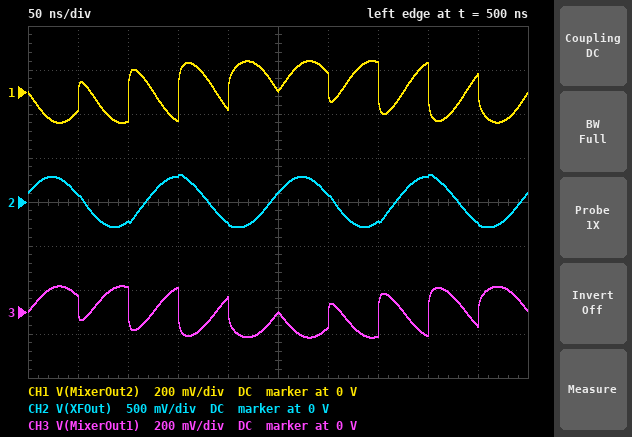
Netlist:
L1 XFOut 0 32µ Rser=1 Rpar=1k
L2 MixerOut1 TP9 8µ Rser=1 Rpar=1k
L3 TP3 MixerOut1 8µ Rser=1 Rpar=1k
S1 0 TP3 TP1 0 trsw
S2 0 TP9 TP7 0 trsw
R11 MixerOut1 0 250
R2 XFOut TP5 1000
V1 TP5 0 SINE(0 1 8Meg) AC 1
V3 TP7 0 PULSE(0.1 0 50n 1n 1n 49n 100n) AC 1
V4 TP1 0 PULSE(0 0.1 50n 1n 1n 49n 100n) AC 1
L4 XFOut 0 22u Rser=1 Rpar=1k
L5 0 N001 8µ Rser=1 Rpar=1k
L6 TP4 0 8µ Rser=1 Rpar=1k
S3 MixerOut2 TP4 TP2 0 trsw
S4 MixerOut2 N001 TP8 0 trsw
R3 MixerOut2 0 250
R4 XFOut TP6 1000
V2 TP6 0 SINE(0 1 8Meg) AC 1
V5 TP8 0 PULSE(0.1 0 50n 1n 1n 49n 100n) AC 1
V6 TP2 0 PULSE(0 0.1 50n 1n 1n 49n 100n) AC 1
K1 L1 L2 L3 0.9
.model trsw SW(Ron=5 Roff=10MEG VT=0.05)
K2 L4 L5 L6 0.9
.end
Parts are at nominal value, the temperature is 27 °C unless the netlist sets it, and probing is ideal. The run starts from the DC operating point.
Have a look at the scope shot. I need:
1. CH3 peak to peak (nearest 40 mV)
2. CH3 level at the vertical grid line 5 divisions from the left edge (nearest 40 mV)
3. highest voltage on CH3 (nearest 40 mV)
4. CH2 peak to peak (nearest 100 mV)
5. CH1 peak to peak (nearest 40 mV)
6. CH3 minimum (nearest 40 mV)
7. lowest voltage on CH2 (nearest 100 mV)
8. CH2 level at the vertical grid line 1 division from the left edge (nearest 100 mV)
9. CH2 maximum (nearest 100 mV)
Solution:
240 mV
0 V
120 mV
600 mV
280 mV
-120 mV
-300 mV
100 mV
300 mV
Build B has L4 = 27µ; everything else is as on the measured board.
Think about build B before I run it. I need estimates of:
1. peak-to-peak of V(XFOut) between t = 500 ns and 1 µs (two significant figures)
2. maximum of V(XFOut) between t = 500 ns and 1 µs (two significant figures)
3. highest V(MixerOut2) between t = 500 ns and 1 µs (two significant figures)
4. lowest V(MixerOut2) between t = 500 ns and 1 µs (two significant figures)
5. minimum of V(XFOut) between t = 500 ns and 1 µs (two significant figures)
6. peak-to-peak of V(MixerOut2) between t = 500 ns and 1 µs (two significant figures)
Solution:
630 mV
330 mV
130 mV
-130 mV
-300 mV
270 mV
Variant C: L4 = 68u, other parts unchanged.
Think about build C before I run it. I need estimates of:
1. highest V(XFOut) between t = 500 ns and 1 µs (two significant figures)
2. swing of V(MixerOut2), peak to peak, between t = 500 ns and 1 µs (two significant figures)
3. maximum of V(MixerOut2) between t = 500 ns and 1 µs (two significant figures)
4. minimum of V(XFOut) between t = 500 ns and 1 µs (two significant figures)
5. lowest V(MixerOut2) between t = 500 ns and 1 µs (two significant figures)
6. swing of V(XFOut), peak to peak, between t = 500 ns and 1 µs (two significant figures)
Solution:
370 mV
200 mV
98 mV
-350 mV
-98 mV
720 mV
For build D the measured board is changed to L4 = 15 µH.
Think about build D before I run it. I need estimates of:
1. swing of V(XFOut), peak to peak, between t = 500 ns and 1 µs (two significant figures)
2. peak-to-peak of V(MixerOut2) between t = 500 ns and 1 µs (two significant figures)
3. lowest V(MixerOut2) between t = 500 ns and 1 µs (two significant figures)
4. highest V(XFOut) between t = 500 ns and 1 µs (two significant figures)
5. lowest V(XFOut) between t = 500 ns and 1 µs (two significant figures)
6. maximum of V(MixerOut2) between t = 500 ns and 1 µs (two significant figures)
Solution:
540 mV
300 mV
-150 mV
280 mV
-260 mV
150 mV
